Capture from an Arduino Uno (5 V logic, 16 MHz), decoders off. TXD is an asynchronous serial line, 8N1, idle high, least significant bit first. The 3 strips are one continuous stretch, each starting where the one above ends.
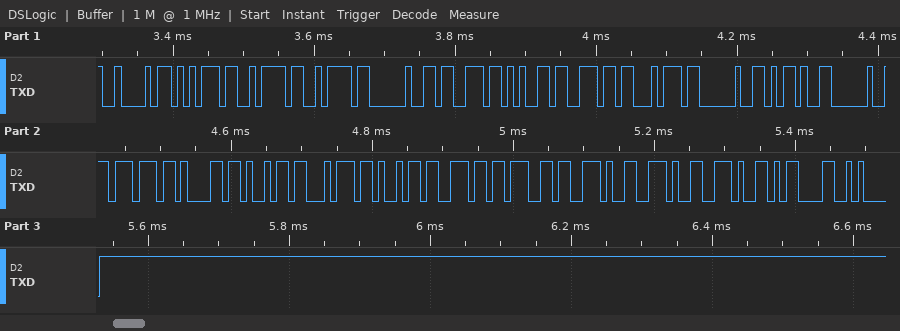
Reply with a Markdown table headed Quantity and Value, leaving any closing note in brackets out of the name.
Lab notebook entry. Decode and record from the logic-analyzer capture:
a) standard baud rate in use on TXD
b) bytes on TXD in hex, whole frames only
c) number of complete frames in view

| Quantity | Value |
|---|---|
| standard baud rate in use on TXD | 115200 baud |
| bytes on TXD in hex, whole frames only | 0x42 0x75 0x7A 0x7A 0x20 0x73 0x65 0x6E 0x74 0x20 0x2D 0x20 0x77 0x61 0x69 0x74 0x69 0x6E 0x67 0x2E 0x2E 0x2E 0x0D 0x0A |
| number of complete frames in view | 24 |
